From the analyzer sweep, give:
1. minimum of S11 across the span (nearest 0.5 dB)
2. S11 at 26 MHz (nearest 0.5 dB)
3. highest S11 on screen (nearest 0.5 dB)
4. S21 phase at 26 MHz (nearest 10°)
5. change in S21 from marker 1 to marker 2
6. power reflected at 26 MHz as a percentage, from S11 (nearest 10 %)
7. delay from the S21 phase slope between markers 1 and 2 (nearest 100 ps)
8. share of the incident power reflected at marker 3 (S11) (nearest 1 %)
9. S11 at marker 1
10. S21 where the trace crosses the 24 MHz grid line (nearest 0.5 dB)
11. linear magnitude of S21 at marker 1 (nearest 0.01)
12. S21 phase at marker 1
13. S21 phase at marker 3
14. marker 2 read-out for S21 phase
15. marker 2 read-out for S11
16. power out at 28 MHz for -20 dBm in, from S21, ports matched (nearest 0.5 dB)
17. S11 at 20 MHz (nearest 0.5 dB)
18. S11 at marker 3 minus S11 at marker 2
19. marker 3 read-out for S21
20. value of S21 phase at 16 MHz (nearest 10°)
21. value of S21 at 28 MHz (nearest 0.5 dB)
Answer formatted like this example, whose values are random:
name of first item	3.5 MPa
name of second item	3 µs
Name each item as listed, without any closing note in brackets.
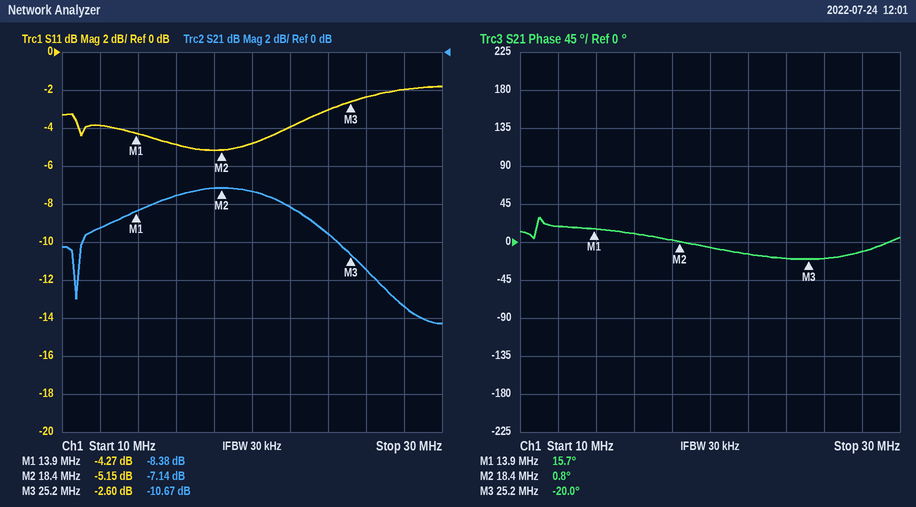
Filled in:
minimum of S11 across the span	-5.0 dB
S11 at 26 MHz	-2.5 dB
highest S11 on screen	-2.0 dB
S21 phase at 26 MHz	-20°
change in S21 from marker 1 to marker 2	1.24 dB
power reflected at 26 MHz as a percentage, from S11	60 %
delay from the S21 phase slope between markers 1 and 2	9.2 ns
share of the incident power reflected at marker 3 (S11)	55 %
S11 at marker 1	-4.27 dB
S21 where the trace crosses the 24 MHz grid line	-9.5 dB
linear magnitude of S21 at marker 1	0.38
S21 phase at marker 1	15.7°
S21 phase at marker 3	-20.0°
marker 2 read-out for S21 phase	0.8°
marker 2 read-out for S11	-5.15 dB
power out at 28 MHz for -20 dBm in, from S21, ports matched	-33.5 dBm
S11 at 20 MHz	-5.0 dB
S11 at marker 3 minus S11 at marker 2	2.55 dB
marker 3 read-out for S21	-10.67 dB
value of S21 phase at 16 MHz	10°
value of S21 at 28 MHz	-13.5 dB
